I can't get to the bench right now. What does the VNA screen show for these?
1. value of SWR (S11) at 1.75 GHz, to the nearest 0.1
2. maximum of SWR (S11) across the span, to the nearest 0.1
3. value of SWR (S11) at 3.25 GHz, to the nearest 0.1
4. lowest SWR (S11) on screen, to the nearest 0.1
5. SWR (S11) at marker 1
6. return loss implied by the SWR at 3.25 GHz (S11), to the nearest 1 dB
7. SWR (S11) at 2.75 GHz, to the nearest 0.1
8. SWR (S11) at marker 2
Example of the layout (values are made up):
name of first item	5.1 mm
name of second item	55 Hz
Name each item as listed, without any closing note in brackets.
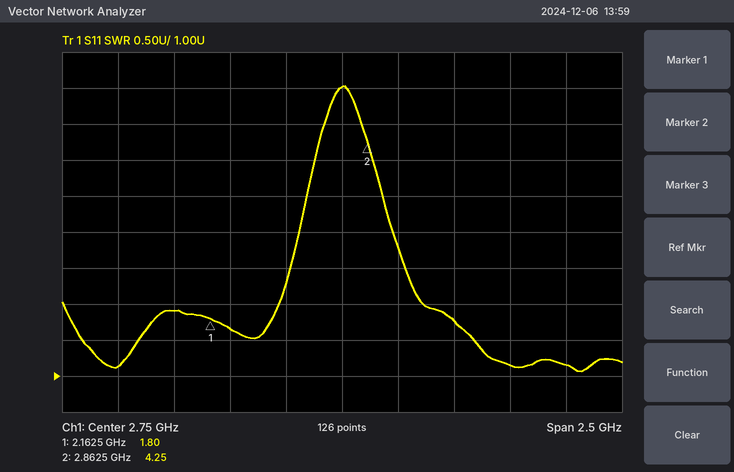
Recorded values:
value of SWR (S11) at 1.75 GHz, to the nearest 0.1	1.1
maximum of SWR (S11) across the span, to the nearest 0.1	5.0
value of SWR (S11) at 3.25 GHz, to the nearest 0.1	1.8
lowest SWR (S11) on screen, to the nearest 0.1	1.1
SWR (S11) at marker 1	1.80
return loss implied by the SWR at 3.25 GHz (S11), to the nearest 1 dB	11 dB
SWR (S11) at 2.75 GHz, to the nearest 0.1	5.0
SWR (S11) at marker 2	4.25
